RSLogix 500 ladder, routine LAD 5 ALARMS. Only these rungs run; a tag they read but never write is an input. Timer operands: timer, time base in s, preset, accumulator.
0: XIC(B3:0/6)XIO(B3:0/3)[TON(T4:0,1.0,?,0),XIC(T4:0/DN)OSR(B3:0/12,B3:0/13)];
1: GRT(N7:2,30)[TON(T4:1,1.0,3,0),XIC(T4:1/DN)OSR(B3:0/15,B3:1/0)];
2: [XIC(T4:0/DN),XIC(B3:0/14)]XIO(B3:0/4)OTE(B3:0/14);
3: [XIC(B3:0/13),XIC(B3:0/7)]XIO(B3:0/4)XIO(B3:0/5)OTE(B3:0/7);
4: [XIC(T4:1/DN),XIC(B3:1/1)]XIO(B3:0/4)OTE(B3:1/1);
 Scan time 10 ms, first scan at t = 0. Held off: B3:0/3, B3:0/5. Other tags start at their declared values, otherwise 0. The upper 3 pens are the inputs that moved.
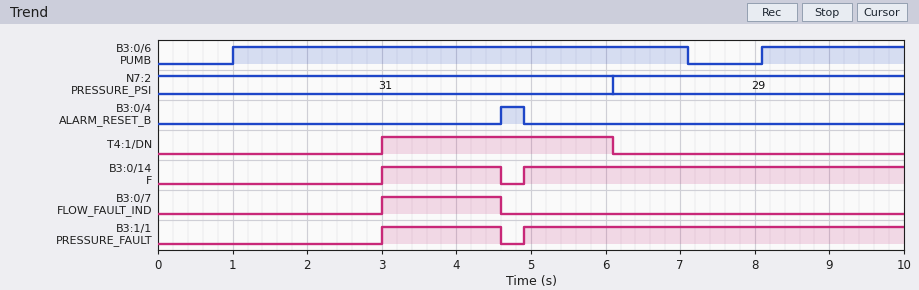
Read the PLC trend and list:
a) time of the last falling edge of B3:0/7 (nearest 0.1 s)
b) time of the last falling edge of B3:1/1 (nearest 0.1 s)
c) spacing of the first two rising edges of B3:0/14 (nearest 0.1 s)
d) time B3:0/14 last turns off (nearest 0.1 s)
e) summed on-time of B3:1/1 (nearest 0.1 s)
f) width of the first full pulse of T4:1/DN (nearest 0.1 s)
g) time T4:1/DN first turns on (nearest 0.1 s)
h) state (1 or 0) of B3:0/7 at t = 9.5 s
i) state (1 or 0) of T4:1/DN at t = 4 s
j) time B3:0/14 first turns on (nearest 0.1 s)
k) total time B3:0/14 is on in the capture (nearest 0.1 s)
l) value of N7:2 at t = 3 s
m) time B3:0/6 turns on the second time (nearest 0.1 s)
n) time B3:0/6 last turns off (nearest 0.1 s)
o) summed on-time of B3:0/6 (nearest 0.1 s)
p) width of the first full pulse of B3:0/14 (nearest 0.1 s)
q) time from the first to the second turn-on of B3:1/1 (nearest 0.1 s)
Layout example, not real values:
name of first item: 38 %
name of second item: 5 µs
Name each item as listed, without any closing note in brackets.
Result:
time of the last falling edge of B3:0/7: 4.6 s
time of the last falling edge of B3:1/1: 4.6 s
spacing of the first two rising edges of B3:0/14: 1.9 s
time B3:0/14 last turns off: 4.6 s
summed on-time of B3:1/1: 6.7 s
width of the first full pulse of T4:1/DN: 3.1 s
time T4:1/DN first turns on: 3.0 s
state (1 or 0) of B3:0/7 at t = 9.5 s: 0
state (1 or 0) of T4:1/DN at t = 4 s: 1
time B3:0/14 first turns on: 3.0 s
total time B3:0/14 is on in the capture: 6.7 s
value of N7:2 at t = 3 s: 31
time B3:0/6 turns on the second time: 8.1 s
time B3:0/6 last turns off: 7.1 s
summed on-time of B3:0/6: 8.0 s
width of the first full pulse of B3:0/14: 1.6 s
time from the first to the second turn-on of B3:1/1: 1.9 s
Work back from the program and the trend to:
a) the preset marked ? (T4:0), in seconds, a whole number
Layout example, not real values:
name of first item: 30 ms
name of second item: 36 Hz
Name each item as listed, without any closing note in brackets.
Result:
the preset marked ? (T4:0), in seconds, a whole number: 2 s
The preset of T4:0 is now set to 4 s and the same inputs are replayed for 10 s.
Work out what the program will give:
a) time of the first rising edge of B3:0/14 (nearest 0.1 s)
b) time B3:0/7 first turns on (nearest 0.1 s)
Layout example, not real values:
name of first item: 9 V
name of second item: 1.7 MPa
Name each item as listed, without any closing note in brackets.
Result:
time of the first rising edge of B3:0/14: 5.0 s
time B3:0/7 first turns on: 5.0 s
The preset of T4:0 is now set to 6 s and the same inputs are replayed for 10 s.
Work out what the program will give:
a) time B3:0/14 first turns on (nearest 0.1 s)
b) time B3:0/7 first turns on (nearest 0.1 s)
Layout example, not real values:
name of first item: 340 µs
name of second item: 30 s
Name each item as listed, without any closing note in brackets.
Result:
time B3:0/14 first turns on: 7.0 s
time B3:0/7 first turns on: 7.0 s
